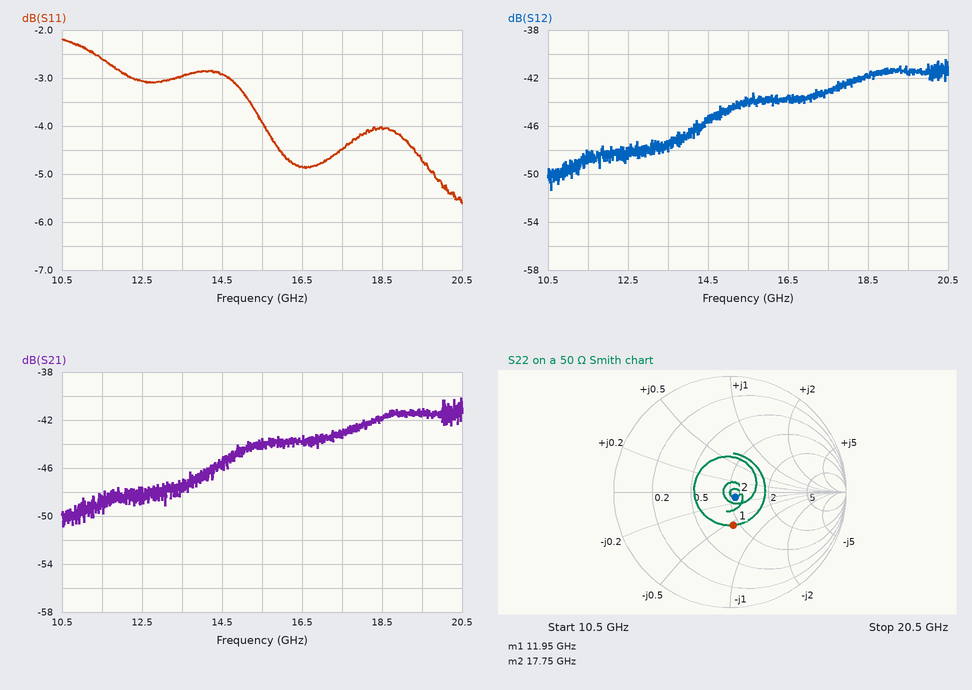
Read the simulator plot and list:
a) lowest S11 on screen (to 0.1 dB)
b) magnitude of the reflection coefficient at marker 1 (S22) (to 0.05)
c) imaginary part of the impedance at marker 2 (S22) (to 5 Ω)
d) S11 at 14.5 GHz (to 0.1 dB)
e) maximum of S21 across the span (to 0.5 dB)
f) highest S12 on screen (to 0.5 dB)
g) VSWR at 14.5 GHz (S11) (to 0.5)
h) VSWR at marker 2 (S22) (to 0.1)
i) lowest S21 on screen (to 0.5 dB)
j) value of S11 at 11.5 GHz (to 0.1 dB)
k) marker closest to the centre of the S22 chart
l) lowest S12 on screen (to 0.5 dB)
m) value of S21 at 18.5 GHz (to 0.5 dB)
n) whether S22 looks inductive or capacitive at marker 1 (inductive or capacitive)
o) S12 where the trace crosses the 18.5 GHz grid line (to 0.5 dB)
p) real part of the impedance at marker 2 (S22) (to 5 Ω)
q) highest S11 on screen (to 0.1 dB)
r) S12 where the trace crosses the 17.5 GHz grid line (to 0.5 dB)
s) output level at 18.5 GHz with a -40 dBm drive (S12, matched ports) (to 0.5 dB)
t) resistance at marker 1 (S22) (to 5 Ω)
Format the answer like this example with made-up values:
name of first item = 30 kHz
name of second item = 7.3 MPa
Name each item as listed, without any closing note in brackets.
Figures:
lowest S11 on screen = -5.6 dB
magnitude of the reflection coefficient at marker 1 (S22) = 0.30
imaginary part of the impedance at marker 2 (S22) = -5 Ω
S11 at 14.5 GHz = -2.9 dB
maximum of S21 across the span = -40.0 dB
highest S12 on screen = -40.5 dB
VSWR at 14.5 GHz (S11) = 6.0
VSWR at marker 2 (S22) = 1.1
lowest S21 on screen = -51.0 dB
value of S11 at 11.5 GHz = -2.6 dB
marker closest to the centre of the S22 chart = marker 2
lowest S12 on screen = -51.5 dB
value of S21 at 18.5 GHz = -42.0 dB
whether S22 looks inductive or capacitive at marker 1 = capacitive
S12 where the trace crosses the 18.5 GHz grid line = -42.0 dB
real part of the impedance at marker 2 (S22) = 55 Ω
highest S11 on screen = -2.2 dB
S12 where the trace crosses the 17.5 GHz grid line = -43.0 dB
output level at 18.5 GHz with a -40 dBm drive (S12, matched ports) = -82.0 dBm
resistance at marker 1 (S22) = 45 Ω
